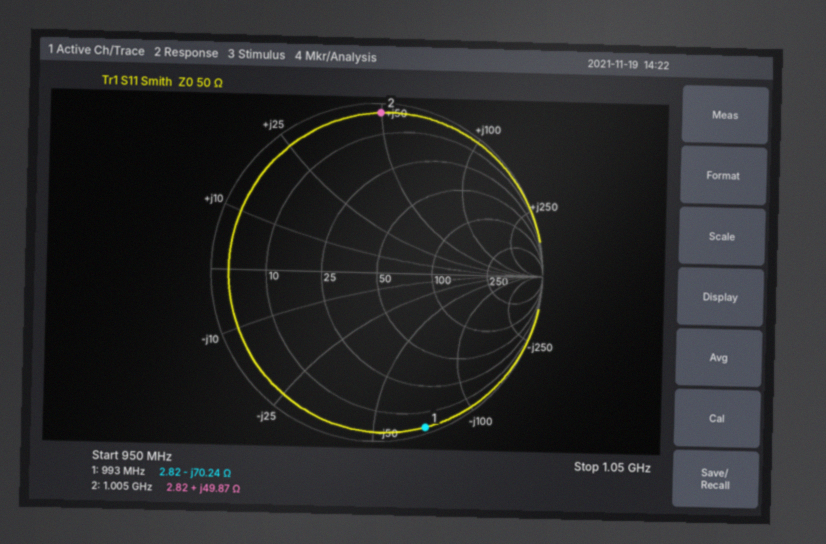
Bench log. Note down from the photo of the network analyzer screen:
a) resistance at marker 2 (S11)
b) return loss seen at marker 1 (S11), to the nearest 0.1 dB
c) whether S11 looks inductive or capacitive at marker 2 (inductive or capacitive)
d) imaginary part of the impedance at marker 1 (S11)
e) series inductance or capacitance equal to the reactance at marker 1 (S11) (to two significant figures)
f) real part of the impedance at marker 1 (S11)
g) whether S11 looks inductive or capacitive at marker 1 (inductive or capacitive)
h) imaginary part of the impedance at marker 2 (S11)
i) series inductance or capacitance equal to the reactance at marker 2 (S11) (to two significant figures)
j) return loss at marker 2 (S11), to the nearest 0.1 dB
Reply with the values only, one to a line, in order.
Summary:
2.82 Ω
0.3 dB
inductive
-70.24 Ω
2.3 pF
2.82 Ω
capacitive
+49.87 Ω
7.9 nH
0.5 dB
